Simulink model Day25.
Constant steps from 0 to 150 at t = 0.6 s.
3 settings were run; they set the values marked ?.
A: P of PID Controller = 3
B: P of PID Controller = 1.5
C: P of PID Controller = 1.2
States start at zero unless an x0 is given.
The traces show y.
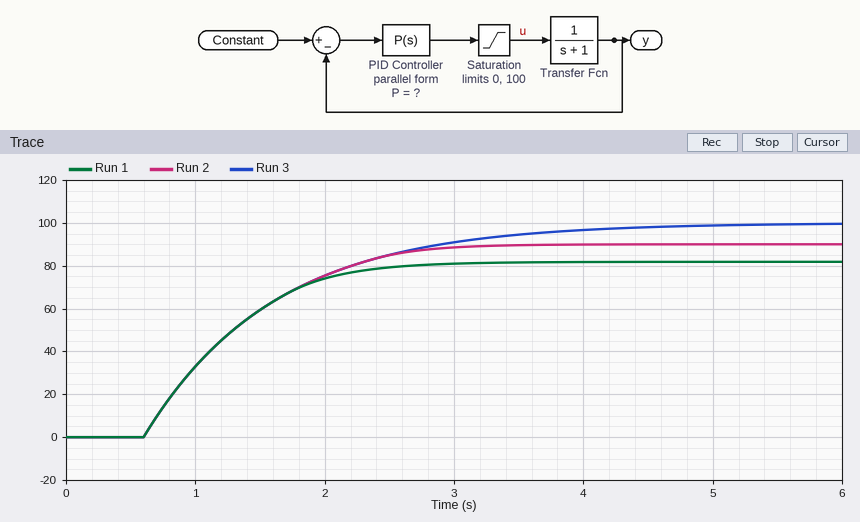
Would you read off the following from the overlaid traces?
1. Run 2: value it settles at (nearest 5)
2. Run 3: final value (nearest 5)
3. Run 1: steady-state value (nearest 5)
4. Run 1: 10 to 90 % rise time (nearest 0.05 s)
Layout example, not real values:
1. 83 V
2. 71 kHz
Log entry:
1. 90
2. 100
3. 80
4. 1.30 s
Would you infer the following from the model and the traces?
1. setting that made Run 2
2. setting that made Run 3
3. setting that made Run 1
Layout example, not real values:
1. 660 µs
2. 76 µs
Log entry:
1. B
2. A
3. C
